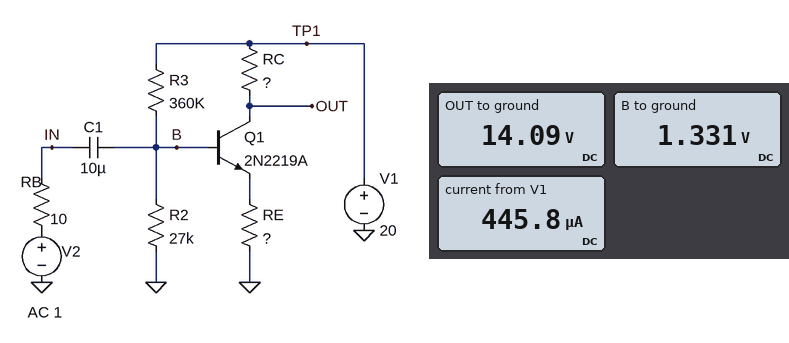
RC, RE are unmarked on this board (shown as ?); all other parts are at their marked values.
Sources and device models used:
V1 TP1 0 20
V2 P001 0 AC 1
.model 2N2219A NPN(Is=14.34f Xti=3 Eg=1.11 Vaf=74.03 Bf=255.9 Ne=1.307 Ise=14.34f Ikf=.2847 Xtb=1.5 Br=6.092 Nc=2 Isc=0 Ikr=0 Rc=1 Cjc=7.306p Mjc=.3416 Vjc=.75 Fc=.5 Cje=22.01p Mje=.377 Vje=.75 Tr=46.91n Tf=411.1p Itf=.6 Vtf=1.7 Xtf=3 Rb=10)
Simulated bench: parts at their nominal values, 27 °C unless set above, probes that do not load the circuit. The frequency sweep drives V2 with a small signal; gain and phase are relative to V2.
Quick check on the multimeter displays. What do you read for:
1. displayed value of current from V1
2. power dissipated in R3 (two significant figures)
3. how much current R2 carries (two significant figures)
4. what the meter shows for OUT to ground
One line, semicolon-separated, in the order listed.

445.8 µA; 970 µW; 49 µA; 14.09 V
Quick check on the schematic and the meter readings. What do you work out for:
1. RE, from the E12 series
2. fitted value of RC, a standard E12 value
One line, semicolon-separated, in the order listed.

1.8 kΩ; 15 kΩ
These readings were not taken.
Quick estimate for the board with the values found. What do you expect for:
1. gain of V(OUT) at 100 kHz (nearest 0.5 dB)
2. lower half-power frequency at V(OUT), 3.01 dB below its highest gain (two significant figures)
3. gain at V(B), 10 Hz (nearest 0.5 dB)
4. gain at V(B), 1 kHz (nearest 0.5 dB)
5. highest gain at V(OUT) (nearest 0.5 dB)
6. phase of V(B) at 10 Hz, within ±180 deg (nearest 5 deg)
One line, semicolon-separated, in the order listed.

18.0 dB; 690 mHz; 0 dB; 0 dB; 18.0 dB; 5 deg
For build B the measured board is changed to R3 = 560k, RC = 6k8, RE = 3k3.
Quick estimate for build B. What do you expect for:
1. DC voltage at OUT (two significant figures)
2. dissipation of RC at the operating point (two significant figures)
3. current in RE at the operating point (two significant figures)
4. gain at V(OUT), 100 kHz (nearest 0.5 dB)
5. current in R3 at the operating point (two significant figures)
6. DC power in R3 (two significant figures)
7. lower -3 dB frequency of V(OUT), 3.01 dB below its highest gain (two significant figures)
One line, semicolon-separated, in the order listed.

19 V; 64 µW; 98 µA; 5.5 dB; 34 µA; 650 µW; 650 mHz
